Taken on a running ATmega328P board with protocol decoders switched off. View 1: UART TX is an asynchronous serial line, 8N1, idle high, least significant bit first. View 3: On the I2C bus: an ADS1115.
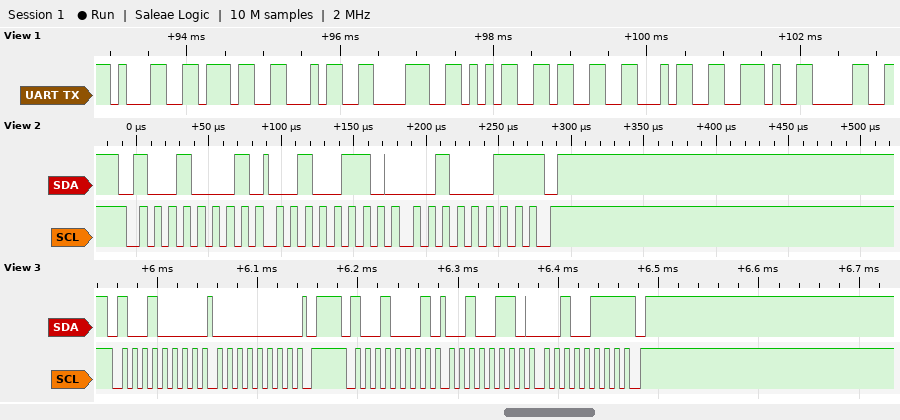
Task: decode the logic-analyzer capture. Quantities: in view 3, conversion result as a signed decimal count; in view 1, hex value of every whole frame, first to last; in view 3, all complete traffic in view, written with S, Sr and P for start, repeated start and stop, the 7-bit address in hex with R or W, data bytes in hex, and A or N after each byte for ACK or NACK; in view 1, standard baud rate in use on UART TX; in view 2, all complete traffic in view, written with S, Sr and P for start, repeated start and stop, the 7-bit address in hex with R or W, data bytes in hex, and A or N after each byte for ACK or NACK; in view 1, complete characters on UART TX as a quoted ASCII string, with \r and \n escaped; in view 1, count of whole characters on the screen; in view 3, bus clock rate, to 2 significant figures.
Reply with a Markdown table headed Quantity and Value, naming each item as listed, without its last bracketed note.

| Quantity | Value |
|---|---|
| in view 3, conversion result as a signed decimal count | 9767 |
| in view 1, hex value of every whole frame, first to last | 31 37 34 38 35 33 34 2E 30 |
| in view 3, all complete traffic in view, written with S, Sr and P for start, repeated start and stop, the 7-bit address in hex with R or W, data bytes in hex, and A or N after each byte for ACK or NACK | S 48W A 00 A P S 48R A 26 A 27 N P |
| in view 1, standard baud rate in use on UART TX | 9600 baud |
| in view 2, all complete traffic in view, written with S, Sr and P for start, repeated start and stop, the 7-bit address in hex with R or W, data bytes in hex, and A or N after each byte for ACK or NACK | S 48R A 26 A 23 N P |
| in view 1, complete characters on UART TX as a quoted ASCII string, with \r and \n escaped | "1748534.0" |
| in view 1, count of whole characters on the screen | 9 |
| in view 3, bus clock rate, to 2 significant figures | 100 kHz |
